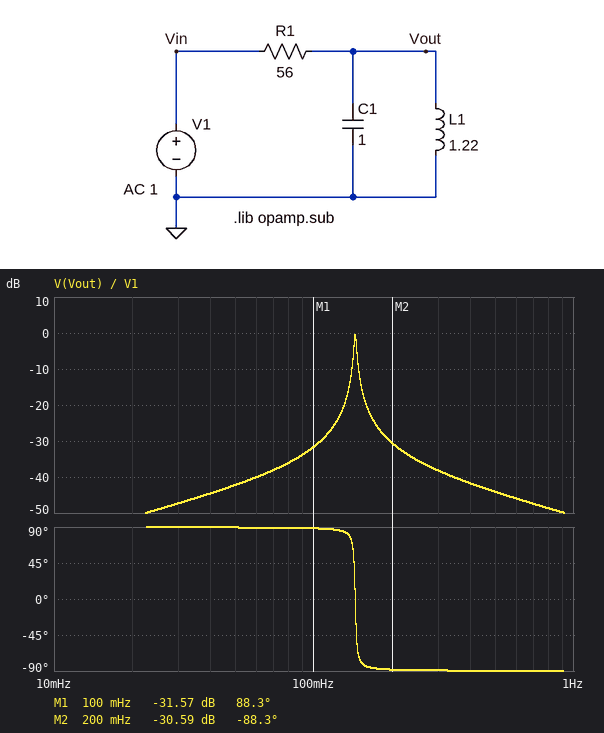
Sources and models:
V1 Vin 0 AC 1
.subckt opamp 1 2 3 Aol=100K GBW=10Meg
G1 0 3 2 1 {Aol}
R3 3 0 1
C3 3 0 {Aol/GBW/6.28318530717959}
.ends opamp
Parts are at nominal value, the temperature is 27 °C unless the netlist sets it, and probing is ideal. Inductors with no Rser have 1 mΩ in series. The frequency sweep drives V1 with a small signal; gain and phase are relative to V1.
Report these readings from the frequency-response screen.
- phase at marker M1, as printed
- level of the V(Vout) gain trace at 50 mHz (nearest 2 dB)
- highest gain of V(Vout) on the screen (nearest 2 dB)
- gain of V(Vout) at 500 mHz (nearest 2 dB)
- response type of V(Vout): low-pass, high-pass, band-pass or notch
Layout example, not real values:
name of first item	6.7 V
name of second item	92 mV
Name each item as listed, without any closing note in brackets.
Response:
phase at marker M1, as printed	88.3 deg
level of the V(Vout) gain trace at 50 mHz	-42 dB
highest gain of V(Vout) on the screen	0 dB
gain of V(Vout) at 500 mHz	-44 dB
response type of V(Vout): low-pass, high-pass, band-pass or notch	band-pass
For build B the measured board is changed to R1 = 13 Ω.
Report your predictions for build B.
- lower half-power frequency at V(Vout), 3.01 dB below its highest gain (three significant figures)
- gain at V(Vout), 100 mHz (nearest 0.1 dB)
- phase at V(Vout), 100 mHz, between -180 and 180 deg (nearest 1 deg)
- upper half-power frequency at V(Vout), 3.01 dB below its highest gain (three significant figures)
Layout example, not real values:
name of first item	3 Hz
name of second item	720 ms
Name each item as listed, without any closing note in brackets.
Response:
lower half-power frequency at V(Vout), 3.01 dB below its highest gain	138 mHz
gain at V(Vout), 100 mHz	-18.9 dB
phase at V(Vout), 100 mHz, between -180 and 180 deg	83 deg
upper half-power frequency at V(Vout), 3.01 dB below its highest gain	150 mHz
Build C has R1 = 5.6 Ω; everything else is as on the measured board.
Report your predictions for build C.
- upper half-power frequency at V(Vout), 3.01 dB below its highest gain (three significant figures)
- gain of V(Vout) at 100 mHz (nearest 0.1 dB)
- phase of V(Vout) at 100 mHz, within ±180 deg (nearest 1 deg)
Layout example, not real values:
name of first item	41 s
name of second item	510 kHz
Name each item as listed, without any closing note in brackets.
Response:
upper half-power frequency at V(Vout), 3.01 dB below its highest gain	159 mHz
gain of V(Vout) at 100 mHz	-11.9 dB
phase of V(Vout) at 100 mHz, within ±180 deg	75 deg
